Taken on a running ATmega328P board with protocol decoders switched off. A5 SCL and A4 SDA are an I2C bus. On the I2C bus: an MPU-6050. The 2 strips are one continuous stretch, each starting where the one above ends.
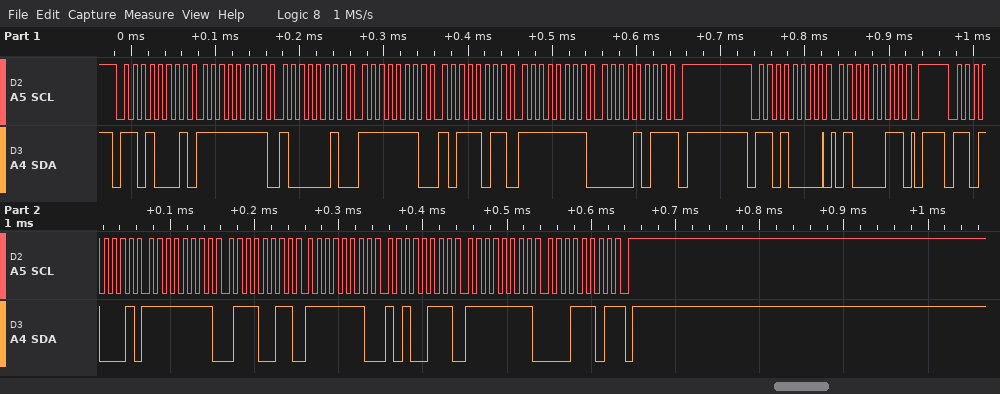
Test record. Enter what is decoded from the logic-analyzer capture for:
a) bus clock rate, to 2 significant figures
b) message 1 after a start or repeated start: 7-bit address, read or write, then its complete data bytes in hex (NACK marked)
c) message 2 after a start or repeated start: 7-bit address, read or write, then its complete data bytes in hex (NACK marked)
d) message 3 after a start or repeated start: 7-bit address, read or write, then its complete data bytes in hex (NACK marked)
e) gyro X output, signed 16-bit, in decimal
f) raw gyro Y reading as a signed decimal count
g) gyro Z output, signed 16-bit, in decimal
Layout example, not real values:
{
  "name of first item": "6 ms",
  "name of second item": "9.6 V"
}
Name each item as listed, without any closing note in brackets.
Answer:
{
  "bus clock rate, to 2 significant figures": "100 kHz",
  "message 1 after a start or repeated start: 7-bit address, read or write, then its complete data bytes in hex": "0x68 read: FF 82 FE BB FF 0B NACK",
  "message 2 after a start or repeated start: 7-bit address, read or write, then its complete data bytes in hex": "0x68 write: 43",
  "message 3 after a start or repeated start: 7-bit address, read or write, then its complete data bytes in hex": "0x68 read: FF 73 FE A7 FF 1D NACK",
  "gyro X output, signed 16-bit, in decimal": "-141",
  "raw gyro Y reading as a signed decimal count": "-345",
  "gyro Z output, signed 16-bit, in decimal": "-227"
}
